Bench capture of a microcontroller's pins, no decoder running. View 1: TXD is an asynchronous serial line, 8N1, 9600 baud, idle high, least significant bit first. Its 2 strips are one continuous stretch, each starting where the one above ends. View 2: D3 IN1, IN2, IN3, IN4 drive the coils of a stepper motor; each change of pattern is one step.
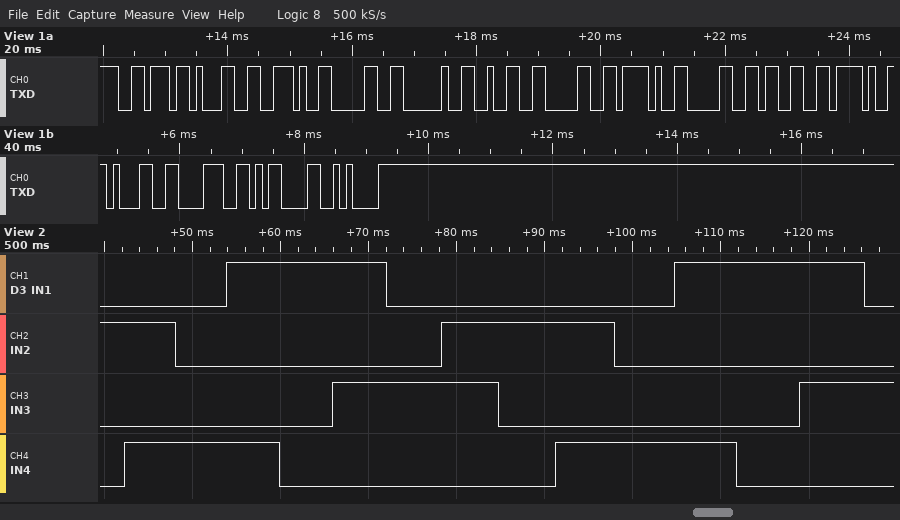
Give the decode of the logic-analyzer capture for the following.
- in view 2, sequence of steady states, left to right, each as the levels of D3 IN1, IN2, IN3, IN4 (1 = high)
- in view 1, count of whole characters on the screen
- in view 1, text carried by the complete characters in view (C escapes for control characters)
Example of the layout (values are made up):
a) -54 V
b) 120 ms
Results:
a) 0100 0101 0001 1001 1000 1010 0010 0110 0100 0101 0001 1001 1000 1010 0010
b) 15
c) "v1.0 20/03/18\r\n"
